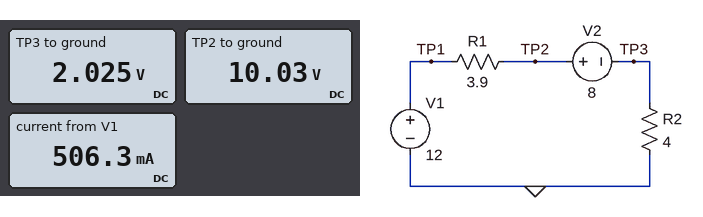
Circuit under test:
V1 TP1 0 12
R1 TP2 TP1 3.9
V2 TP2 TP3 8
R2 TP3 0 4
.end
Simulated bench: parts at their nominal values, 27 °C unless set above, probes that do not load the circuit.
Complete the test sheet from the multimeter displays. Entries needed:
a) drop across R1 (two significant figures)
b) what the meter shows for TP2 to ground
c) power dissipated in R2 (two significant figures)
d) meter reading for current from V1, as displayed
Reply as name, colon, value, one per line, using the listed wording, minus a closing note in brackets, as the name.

drop across R1: 2.0 V
what the meter shows for TP2 to ground: 10.03 V
power dissipated in R2: 1.0 W
meter reading for current from V1, as displayed: 506.3 mA
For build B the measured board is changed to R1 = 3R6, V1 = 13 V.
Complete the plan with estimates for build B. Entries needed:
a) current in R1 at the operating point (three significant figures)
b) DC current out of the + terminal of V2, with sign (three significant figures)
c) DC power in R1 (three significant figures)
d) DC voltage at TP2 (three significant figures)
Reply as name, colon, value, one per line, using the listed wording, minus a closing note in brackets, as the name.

current in R1 at the operating point: 658 mA
DC current out of the + terminal of V2, with sign: -658 mA
DC power in R1: 1.56 W
DC voltage at TP2: 10.6 V
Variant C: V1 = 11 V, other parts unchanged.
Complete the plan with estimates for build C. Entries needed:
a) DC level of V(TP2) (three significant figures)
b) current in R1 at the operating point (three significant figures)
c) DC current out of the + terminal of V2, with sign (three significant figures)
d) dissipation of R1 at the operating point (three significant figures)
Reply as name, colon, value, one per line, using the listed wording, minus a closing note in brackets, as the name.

DC level of V(TP2): 9.52 V
current in R1 at the operating point: 380 mA
DC current out of the + terminal of V2, with sign: -380 mA
dissipation of R1 at the operating point: 562 mW
